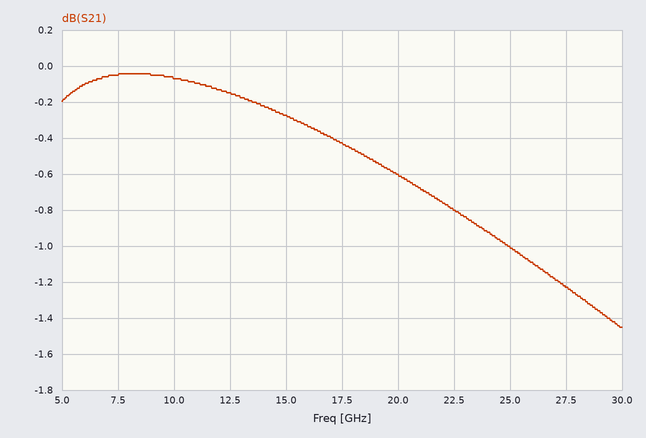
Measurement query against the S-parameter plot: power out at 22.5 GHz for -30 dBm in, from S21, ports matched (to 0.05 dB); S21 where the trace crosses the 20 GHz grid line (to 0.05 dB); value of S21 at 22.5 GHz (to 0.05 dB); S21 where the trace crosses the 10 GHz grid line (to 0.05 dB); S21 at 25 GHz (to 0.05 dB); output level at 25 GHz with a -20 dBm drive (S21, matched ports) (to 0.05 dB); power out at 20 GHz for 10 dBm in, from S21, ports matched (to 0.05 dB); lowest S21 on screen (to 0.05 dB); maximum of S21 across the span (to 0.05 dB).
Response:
-30.80 dBm
-0.60 dB
-0.80 dB
-0.05 dB
-1.00 dB
-21.00 dBm
9.40 dBm
-1.45 dB
-0.05 dB
